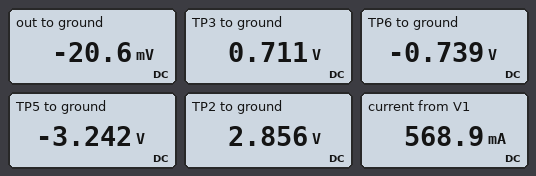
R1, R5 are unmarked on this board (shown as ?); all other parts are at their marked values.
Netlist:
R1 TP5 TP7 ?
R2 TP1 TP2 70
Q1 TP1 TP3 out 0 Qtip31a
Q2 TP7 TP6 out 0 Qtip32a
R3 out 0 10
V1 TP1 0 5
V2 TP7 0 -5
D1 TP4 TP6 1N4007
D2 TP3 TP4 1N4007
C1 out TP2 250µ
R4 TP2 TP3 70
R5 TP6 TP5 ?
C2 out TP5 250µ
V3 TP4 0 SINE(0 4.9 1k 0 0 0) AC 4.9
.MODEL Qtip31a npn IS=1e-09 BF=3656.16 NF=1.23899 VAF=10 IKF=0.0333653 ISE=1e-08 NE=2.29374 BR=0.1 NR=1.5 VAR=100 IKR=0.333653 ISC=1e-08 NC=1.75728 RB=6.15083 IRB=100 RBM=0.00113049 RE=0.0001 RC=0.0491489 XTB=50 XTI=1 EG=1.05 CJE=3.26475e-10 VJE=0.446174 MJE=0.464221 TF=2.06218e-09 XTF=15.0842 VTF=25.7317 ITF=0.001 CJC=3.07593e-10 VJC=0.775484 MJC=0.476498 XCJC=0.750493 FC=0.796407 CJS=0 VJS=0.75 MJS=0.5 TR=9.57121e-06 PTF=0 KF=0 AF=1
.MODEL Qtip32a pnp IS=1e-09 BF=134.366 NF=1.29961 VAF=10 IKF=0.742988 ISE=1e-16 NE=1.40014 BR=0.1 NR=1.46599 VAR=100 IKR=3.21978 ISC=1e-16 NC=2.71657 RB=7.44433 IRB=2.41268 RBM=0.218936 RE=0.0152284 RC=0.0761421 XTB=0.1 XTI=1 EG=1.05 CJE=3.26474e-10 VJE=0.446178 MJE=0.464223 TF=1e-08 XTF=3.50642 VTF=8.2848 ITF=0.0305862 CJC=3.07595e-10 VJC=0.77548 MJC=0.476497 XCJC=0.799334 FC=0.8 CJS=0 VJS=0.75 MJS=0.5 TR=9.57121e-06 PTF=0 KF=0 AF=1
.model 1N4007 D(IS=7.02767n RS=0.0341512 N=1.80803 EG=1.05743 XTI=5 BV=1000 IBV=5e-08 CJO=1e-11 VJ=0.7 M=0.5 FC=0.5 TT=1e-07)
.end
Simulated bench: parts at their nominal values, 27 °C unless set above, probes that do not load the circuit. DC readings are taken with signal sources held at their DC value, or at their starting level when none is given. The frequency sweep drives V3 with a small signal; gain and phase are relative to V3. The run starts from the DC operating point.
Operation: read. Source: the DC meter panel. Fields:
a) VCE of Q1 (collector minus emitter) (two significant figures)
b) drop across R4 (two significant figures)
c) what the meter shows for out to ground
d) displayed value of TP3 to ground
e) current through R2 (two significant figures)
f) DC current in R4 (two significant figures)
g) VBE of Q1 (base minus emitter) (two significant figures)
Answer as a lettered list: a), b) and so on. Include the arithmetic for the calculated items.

a) 5 V - (-20.6 mV) = 5.0 V
b) 2.856 V - 711 mV = 2.1 V
c) -20.6 mV
d) 0.711 V
e) (5 V - 2.856 V) / 70 Ω = 31 mA
f) (2.856 V - 711 mV) / 70 Ω = 31 mA
g) 711 mV - (-20.6 mV) = 730 mV
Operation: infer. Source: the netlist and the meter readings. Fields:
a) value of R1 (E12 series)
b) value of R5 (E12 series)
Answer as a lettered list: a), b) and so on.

a) 33 Ω
b) 47 Ω
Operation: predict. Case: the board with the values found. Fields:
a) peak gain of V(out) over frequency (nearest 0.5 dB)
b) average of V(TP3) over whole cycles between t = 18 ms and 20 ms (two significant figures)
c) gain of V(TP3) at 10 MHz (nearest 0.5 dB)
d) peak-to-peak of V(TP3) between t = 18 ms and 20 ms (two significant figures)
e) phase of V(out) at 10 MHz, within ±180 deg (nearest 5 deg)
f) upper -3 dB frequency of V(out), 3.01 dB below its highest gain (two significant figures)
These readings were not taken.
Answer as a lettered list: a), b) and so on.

a) 0 dB
b) 710 mV
c) 0 dB
d) 9.8 V
e) -10 deg
f) 6.4 MHz
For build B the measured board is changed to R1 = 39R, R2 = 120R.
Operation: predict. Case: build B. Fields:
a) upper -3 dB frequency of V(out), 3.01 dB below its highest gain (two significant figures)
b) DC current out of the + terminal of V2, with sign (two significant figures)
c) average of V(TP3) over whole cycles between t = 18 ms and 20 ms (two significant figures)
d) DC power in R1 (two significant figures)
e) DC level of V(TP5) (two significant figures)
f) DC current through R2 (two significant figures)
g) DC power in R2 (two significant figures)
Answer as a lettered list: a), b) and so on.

a) 7.7 MHz
b) -540 mA
c) 690 mV
d) 96 mW
e) -3.1 V
f) 23 mA
g) 62 mW
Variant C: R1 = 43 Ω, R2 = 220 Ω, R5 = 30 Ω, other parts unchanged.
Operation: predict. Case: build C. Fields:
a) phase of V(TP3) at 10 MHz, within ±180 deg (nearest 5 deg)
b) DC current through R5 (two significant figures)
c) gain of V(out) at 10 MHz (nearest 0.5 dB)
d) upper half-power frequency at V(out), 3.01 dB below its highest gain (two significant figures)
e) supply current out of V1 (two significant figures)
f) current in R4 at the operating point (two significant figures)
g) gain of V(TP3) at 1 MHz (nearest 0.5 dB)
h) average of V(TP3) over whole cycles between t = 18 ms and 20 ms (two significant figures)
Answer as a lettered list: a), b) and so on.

a) 0 deg
b) 58 mA
c) -3.0 dB
d) 9.8 MHz
e) 460 mA
f) 15 mA
g) -0.5 dB
h) 670 mV
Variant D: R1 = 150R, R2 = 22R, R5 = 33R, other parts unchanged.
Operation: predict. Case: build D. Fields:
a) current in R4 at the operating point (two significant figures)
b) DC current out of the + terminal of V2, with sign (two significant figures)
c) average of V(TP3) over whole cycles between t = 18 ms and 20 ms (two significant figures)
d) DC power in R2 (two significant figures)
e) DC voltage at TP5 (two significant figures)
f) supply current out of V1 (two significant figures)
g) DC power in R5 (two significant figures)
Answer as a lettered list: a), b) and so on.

a) 46 mA
b) -500 mA
c) 730 mV
d) 47 mW
e) -1.5 V
f) 530 mA
g) 18 mW
